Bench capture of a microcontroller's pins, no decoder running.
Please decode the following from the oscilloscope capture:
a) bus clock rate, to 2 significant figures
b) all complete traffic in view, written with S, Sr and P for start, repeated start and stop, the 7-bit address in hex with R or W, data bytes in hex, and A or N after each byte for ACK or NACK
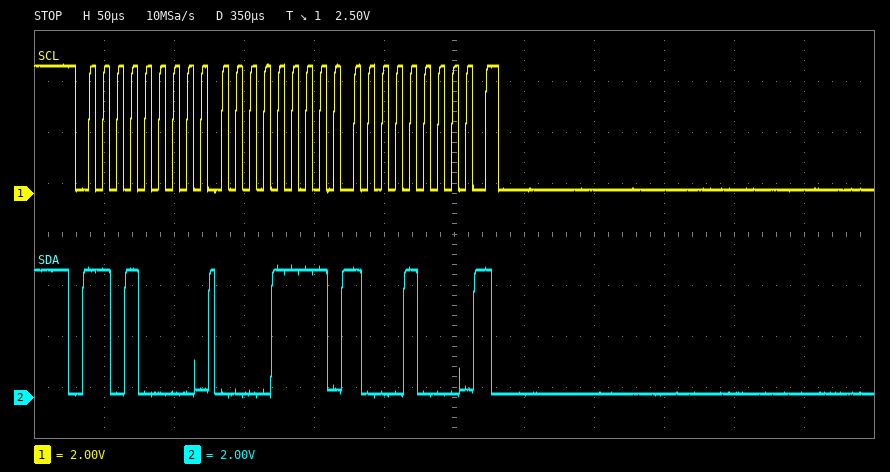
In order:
100 kHz
S 68W A 0F A 88 A
